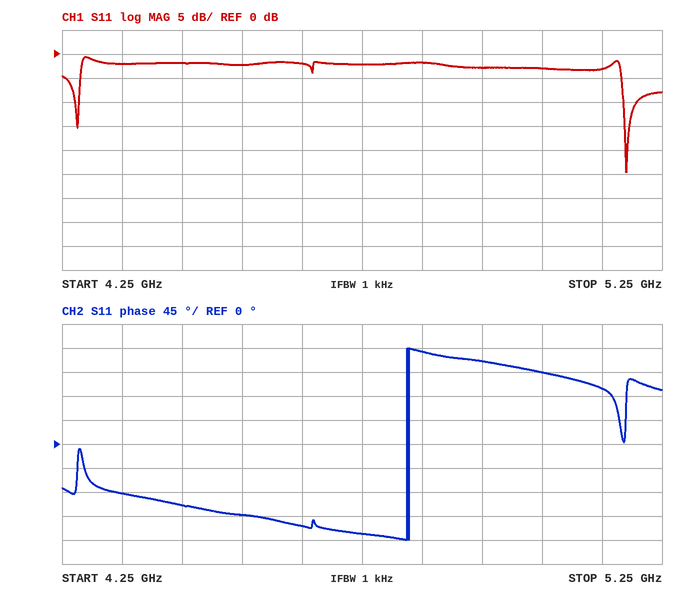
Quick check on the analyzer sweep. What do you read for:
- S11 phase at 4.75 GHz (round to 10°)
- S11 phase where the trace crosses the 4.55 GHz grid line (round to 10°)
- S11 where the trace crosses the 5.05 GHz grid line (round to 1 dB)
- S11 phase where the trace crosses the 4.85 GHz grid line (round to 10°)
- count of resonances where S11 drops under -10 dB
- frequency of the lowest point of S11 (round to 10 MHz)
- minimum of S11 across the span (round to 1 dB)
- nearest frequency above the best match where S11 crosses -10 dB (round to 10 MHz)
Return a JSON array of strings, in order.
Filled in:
["-170°", "-130°", "-3 dB", "170°", "2", "5.19 GHz", "-25 dB", "5.21 GHz"]
